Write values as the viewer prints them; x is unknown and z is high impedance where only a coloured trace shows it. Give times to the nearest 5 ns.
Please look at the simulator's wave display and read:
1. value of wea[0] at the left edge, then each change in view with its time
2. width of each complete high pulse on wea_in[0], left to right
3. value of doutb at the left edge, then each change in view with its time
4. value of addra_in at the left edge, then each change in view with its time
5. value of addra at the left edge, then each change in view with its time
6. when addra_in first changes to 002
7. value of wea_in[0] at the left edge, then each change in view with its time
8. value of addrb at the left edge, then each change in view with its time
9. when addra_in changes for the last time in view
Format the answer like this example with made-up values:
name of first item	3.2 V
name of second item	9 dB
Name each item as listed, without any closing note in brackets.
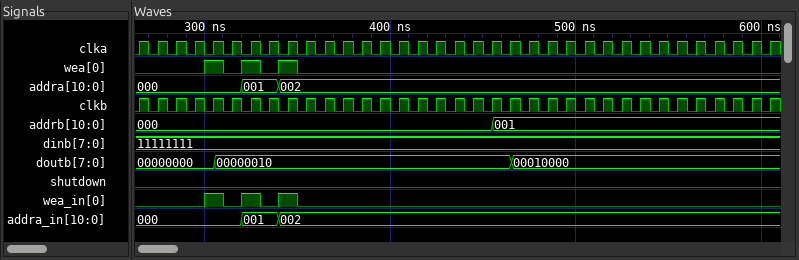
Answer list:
value of wea[0] at the left edge, then each change in view with its time	0, 1 at 300 ns, 0 at 310 ns, 1 at 320 ns, 0 at 330 ns, 1 at 340 ns, 0 at 350 ns
width of each complete high pulse on wea_in[0], left to right	10 ns, 10 ns, 10 ns
value of doutb at the left edge, then each change in view with its time	00000000, 00000010 at 305 ns, 00010000 at 465 ns
value of addra_in at the left edge, then each change in view with its time	000, 001 at 320 ns, 002 at 340 ns
value of addra at the left edge, then each change in view with its time	000, 001 at 320 ns, 002 at 340 ns
when addra_in first changes to 002	340 ns
value of wea_in[0] at the left edge, then each change in view with its time	0, 1 at 300 ns, 0 at 310 ns, 1 at 320 ns, 0 at 330 ns, 1 at 340 ns, 0 at 350 ns
value of addrb at the left edge, then each change in view with its time	000, 001 at 455 ns
when addra_in changes for the last time in view	340 ns
